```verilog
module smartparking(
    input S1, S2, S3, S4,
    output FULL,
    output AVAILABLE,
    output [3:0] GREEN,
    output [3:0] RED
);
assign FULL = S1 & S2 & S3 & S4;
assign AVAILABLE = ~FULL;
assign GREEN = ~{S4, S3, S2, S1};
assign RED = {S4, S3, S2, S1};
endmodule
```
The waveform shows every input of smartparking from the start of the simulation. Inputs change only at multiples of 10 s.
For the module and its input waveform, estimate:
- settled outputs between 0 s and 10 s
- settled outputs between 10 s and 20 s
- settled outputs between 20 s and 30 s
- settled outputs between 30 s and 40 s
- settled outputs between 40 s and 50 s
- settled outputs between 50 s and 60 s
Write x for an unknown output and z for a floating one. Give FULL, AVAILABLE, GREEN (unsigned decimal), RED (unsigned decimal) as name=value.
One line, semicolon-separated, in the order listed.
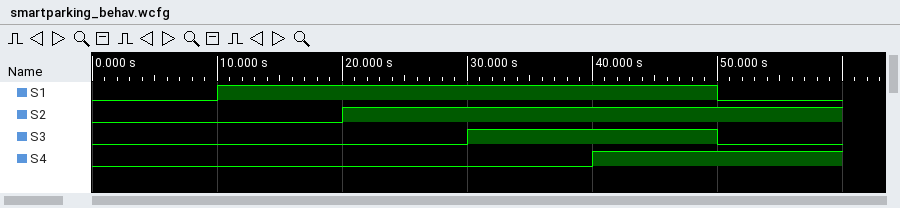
FULL=0, AVAILABLE=1, GREEN=15, RED=0; FULL=0, AVAILABLE=1, GREEN=14, RED=1; FULL=0, AVAILABLE=1, GREEN=12, RED=3; FULL=0, AVAILABLE=1, GREEN=8, RED=7; FULL=1, AVAILABLE=0, GREEN=0, RED=15; FULL=0, AVAILABLE=1, GREEN=5, RED=10
